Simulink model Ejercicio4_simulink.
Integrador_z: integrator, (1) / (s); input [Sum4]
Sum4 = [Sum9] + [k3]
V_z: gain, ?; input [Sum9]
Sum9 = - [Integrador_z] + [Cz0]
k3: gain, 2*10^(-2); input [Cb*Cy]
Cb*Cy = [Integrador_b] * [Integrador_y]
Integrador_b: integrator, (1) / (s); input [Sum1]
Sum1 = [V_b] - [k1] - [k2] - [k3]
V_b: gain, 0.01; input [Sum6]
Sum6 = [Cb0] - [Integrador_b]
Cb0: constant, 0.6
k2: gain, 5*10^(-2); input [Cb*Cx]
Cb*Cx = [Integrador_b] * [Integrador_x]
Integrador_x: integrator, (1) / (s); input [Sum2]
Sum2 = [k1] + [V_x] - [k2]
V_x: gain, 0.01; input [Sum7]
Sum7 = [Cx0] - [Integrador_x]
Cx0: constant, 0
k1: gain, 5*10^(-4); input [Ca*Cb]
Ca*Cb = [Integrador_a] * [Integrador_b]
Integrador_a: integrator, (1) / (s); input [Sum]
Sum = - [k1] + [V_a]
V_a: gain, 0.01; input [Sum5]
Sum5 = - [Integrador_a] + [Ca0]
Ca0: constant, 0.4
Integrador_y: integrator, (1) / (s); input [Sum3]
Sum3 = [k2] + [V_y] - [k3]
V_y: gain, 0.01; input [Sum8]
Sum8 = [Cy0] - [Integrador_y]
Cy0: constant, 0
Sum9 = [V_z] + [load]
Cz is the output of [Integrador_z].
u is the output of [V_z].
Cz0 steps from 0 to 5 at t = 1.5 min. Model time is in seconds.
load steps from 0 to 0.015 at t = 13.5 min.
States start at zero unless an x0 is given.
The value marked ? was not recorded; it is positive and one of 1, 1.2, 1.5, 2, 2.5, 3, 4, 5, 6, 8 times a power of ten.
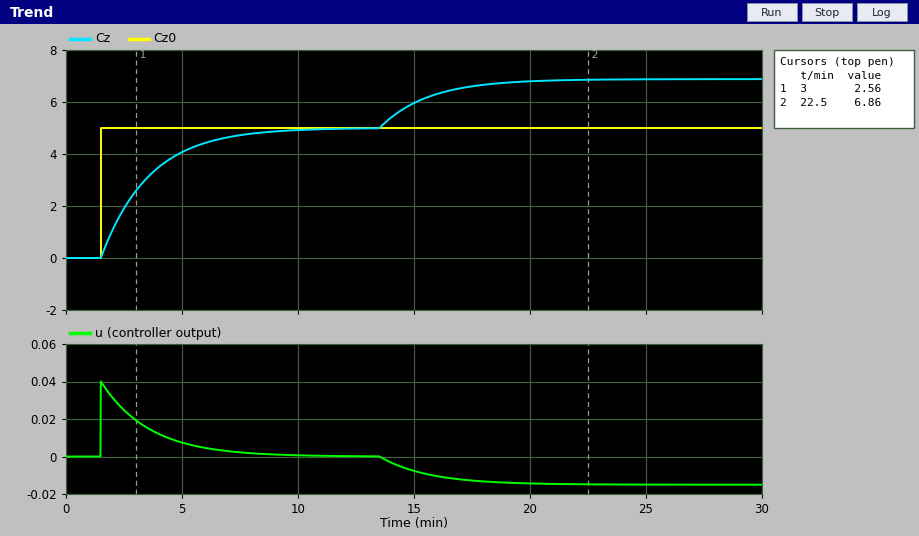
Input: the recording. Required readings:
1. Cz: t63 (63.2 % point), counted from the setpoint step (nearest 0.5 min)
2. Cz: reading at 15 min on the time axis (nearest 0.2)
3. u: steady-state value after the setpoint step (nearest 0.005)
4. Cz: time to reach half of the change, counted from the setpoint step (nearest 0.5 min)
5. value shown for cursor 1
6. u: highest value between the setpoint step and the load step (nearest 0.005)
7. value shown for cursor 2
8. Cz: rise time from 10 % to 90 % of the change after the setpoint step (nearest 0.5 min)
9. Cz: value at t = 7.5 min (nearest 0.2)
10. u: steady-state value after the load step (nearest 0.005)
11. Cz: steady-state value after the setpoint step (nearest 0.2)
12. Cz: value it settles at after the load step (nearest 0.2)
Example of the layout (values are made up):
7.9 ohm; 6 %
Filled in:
2.0 min; 6.0; 0.000; 1.5 min; 2.56; 0.040; 6.86; 4.5 min; 4.8; -0.015; 5.0; 6.8
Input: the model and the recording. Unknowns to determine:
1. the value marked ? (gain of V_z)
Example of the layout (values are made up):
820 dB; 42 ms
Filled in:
0.008
